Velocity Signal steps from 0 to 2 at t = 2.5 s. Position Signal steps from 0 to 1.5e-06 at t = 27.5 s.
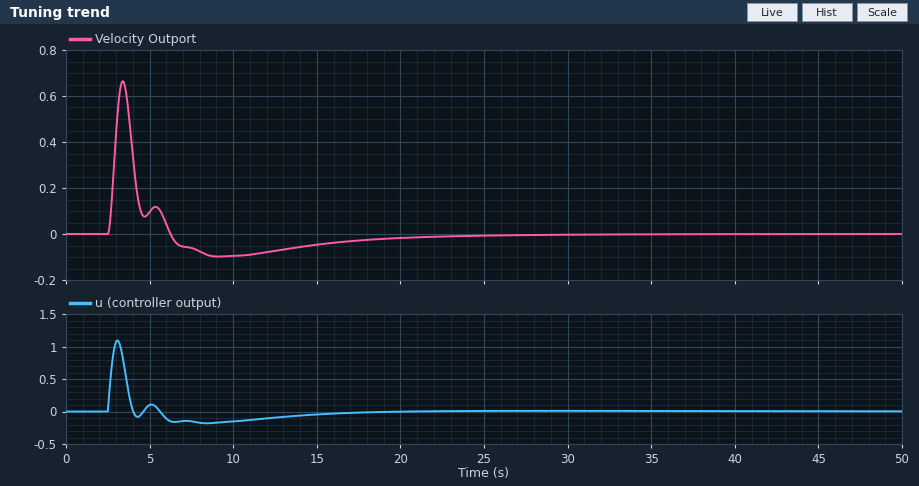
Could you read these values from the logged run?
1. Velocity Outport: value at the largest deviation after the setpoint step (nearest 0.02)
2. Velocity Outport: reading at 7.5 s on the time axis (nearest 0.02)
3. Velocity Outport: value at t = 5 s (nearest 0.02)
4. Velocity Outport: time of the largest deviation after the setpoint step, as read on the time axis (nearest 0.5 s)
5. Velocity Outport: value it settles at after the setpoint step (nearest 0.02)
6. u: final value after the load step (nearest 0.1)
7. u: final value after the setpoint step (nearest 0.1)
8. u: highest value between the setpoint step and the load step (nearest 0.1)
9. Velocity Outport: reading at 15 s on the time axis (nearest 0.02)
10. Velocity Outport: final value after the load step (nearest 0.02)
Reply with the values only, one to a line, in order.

0.66
-0.06
0.10
3.5 s
0.00
0.0
0.0
1.1
-0.04
0.00
